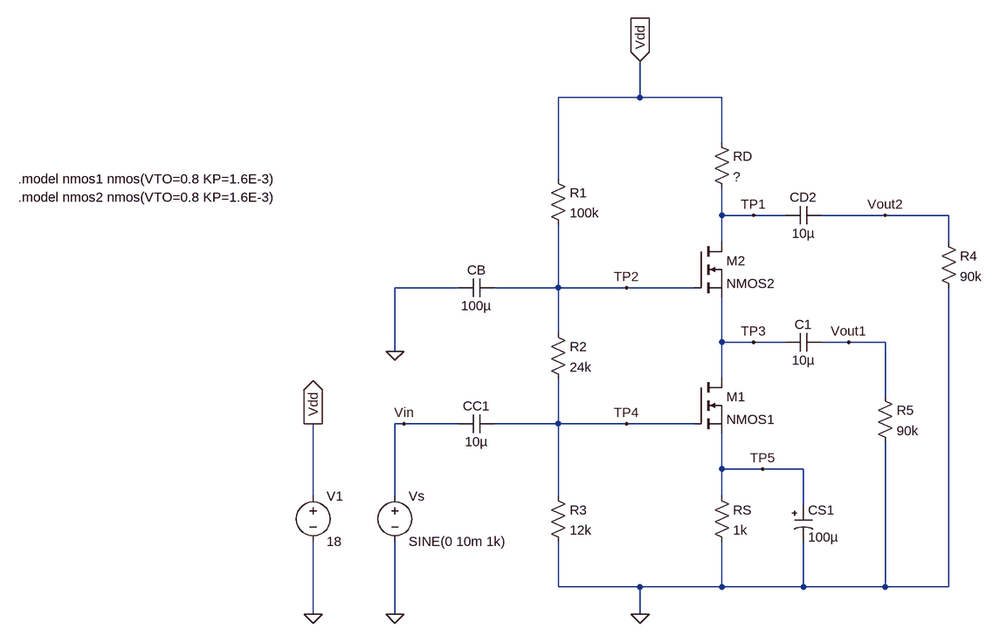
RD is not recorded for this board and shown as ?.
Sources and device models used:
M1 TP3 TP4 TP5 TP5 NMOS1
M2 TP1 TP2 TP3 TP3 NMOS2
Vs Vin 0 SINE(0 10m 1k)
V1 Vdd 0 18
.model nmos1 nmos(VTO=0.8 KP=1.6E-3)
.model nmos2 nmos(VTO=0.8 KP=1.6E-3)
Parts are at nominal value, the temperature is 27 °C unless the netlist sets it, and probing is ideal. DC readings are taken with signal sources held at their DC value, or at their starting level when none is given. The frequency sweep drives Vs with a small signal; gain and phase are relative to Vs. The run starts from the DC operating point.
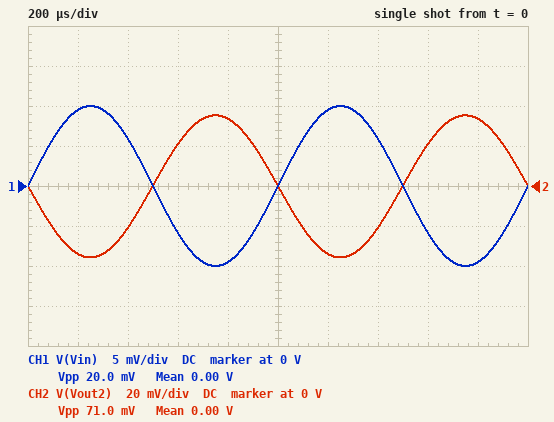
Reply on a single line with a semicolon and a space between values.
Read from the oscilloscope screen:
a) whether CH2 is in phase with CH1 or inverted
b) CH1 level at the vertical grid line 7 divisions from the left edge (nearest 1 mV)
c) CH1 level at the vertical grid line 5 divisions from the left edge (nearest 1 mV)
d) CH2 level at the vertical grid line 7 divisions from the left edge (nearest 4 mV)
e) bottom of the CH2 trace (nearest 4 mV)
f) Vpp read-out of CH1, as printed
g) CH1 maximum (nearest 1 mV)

inverted; 6 mV; 0 V; -20 mV; -36 mV; 20.0 mV; 10 mV
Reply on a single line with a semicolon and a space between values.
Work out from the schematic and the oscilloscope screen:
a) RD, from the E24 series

4.3 kΩ
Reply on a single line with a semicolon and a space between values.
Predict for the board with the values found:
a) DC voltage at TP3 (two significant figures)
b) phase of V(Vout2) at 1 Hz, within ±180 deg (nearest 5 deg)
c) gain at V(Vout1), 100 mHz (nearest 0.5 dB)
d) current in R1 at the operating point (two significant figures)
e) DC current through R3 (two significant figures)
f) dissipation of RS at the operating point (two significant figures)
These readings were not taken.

3.4 V; -95 deg; -38.0 dB; 130 µA; 130 µA; 58 µW
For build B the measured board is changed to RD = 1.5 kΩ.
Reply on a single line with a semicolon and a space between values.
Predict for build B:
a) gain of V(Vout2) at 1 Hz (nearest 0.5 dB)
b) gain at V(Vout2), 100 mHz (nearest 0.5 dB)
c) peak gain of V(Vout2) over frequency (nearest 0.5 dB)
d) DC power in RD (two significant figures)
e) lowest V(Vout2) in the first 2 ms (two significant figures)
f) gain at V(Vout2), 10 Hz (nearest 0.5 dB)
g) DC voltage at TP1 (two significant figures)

-9.5 dB; -34.5 dB; 2.0 dB; 87 µW; -13 mV; 1.5 dB; 18 V
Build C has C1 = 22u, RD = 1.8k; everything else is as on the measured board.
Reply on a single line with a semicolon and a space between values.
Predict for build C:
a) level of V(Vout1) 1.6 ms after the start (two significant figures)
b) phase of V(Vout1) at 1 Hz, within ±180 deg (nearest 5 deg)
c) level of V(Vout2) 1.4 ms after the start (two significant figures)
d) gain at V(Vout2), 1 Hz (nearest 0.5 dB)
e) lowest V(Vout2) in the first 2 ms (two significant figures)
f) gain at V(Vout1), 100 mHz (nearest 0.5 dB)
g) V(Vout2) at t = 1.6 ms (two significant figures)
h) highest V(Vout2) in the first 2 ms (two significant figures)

5.9 mV; -95 deg; -8.9 mV; -8.0 dB; -15 mV; -34.0 dB; 9.0 mV; 15 mV
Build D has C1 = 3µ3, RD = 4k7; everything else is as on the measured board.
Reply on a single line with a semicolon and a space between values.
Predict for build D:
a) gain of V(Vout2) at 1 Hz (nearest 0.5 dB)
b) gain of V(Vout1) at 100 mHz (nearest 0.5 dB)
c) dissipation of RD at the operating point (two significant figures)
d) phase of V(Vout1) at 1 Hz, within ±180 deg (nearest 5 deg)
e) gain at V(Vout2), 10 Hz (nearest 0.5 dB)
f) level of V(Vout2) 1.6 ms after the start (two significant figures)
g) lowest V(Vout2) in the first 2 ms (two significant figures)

0 dB; -46.5 dB; 270 µW; -70 deg; 11.5 dB; 23 mV; -39 mV
